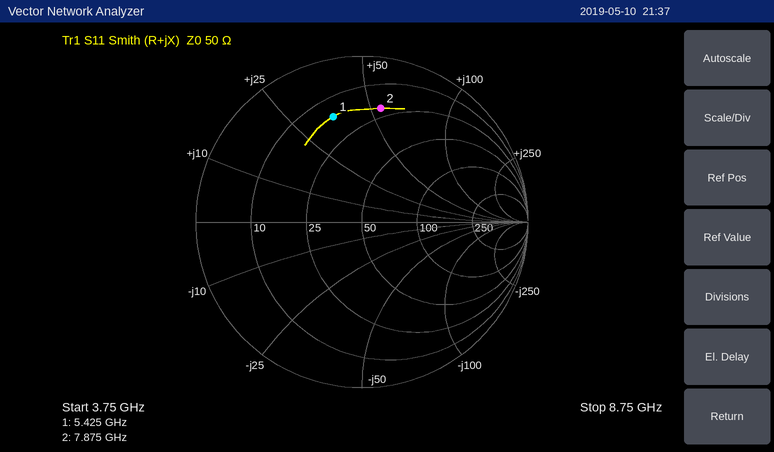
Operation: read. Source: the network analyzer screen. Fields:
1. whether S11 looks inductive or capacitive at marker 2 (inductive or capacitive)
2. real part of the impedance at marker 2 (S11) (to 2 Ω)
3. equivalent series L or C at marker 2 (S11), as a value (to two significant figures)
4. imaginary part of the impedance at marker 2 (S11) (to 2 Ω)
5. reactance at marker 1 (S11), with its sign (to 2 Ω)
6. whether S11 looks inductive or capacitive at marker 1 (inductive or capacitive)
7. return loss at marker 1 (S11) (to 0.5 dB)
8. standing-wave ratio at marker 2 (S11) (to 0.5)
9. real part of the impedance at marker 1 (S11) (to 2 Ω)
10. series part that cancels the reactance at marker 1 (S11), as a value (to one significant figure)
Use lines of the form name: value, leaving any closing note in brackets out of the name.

whether S11 looks inductive or capacitive at marker 2: inductive
real part of the impedance at marker 2 (S11): 20 Ω
equivalent series L or C at marker 2 (S11), as a value: 1.1 nH
imaginary part of the impedance at marker 2 (S11): +54 Ω
reactance at marker 1 (S11), with its sign: +36 Ω
whether S11 looks inductive or capacitive at marker 1: inductive
return loss at marker 1 (S11): 3.5 dB
standing-wave ratio at marker 2 (S11): 5.5
real part of the impedance at marker 1 (S11): 16 Ω
series part that cancels the reactance at marker 1 (S11), as a value: 800 fF
